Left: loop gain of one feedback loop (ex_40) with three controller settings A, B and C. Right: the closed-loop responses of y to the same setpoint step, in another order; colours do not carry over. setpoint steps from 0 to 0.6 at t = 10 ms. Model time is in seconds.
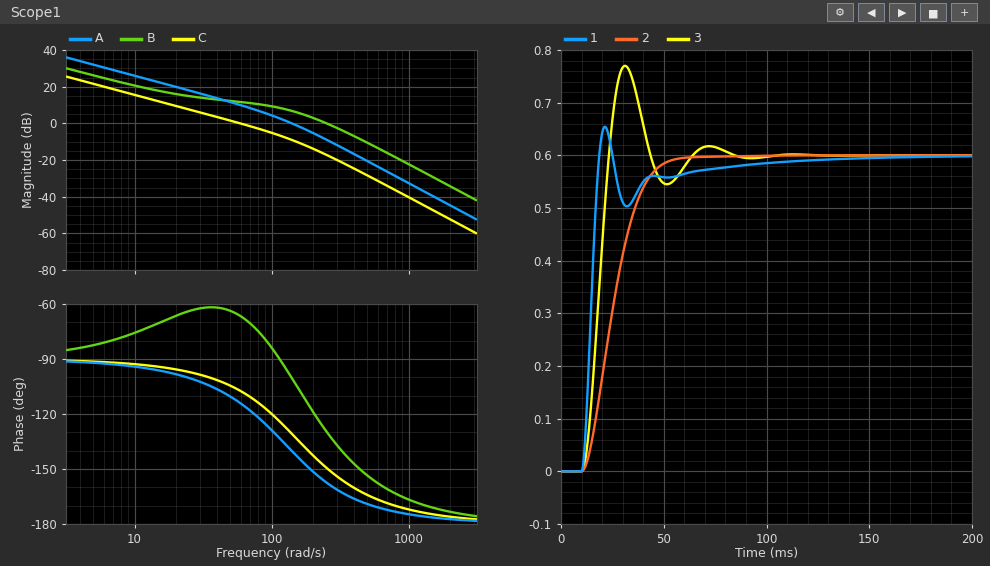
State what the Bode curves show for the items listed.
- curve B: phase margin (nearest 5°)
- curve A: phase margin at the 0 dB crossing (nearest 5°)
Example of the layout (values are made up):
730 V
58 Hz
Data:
50°
40°
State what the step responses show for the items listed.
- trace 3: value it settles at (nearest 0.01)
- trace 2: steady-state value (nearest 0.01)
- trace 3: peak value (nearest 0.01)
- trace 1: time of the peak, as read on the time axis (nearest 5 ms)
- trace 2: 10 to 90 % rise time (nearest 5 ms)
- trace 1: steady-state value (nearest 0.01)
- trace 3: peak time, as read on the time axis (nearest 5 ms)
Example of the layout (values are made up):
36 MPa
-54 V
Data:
0.60
0.60
0.77
20 ms
25 ms
0.60
30 ms
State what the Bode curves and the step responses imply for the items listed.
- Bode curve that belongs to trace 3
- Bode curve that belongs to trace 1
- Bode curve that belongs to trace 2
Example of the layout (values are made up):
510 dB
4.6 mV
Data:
A
B
C
